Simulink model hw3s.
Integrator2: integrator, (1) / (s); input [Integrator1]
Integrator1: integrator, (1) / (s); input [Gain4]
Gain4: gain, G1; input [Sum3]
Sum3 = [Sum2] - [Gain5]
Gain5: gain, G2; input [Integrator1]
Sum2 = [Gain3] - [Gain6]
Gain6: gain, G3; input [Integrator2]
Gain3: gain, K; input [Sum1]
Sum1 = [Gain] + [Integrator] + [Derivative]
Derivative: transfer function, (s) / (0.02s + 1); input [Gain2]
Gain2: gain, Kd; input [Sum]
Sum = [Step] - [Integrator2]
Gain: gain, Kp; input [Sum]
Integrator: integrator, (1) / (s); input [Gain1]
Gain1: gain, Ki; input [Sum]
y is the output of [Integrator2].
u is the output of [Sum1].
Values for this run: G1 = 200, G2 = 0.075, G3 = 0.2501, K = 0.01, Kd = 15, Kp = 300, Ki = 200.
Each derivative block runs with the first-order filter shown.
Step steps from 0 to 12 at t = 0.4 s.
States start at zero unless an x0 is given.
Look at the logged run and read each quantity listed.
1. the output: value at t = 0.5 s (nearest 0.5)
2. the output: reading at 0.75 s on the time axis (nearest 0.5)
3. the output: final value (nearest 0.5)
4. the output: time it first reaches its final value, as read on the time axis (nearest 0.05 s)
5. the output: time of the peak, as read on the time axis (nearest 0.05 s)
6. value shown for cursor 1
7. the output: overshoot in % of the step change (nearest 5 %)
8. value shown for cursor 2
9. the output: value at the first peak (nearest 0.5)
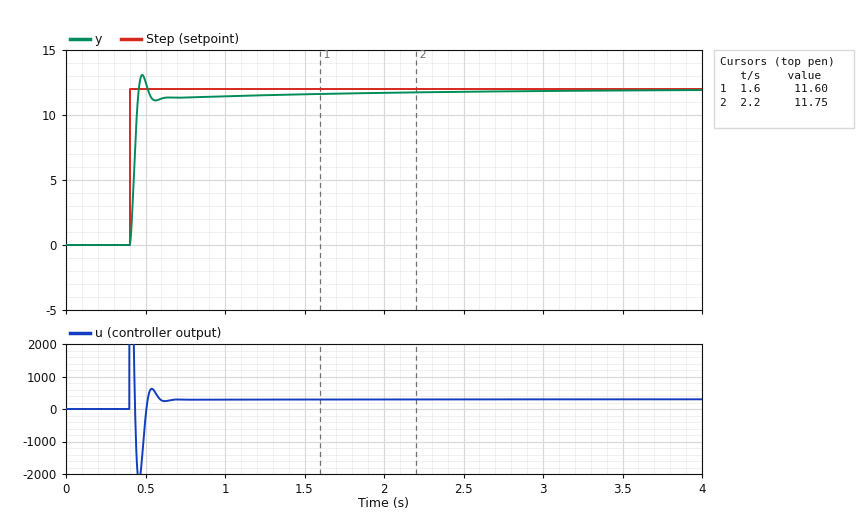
12.5
11.5
12.0
0.45 s
0.50 s
11.60
10 %
11.75
13.0
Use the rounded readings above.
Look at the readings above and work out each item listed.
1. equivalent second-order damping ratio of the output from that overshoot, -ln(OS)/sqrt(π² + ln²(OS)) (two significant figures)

0.59
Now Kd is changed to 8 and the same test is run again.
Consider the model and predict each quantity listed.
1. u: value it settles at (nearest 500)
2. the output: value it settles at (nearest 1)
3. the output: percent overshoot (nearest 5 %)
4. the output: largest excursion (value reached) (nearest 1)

500
12
15 %
14
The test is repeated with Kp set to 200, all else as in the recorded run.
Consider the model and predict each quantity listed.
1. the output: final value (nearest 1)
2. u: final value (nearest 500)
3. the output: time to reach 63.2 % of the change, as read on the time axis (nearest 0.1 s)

12
500
0.4 s
